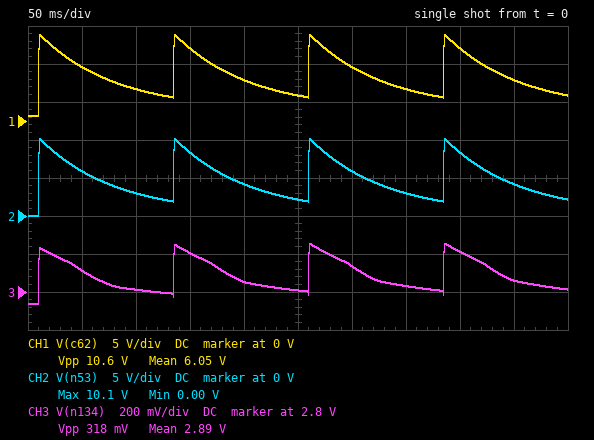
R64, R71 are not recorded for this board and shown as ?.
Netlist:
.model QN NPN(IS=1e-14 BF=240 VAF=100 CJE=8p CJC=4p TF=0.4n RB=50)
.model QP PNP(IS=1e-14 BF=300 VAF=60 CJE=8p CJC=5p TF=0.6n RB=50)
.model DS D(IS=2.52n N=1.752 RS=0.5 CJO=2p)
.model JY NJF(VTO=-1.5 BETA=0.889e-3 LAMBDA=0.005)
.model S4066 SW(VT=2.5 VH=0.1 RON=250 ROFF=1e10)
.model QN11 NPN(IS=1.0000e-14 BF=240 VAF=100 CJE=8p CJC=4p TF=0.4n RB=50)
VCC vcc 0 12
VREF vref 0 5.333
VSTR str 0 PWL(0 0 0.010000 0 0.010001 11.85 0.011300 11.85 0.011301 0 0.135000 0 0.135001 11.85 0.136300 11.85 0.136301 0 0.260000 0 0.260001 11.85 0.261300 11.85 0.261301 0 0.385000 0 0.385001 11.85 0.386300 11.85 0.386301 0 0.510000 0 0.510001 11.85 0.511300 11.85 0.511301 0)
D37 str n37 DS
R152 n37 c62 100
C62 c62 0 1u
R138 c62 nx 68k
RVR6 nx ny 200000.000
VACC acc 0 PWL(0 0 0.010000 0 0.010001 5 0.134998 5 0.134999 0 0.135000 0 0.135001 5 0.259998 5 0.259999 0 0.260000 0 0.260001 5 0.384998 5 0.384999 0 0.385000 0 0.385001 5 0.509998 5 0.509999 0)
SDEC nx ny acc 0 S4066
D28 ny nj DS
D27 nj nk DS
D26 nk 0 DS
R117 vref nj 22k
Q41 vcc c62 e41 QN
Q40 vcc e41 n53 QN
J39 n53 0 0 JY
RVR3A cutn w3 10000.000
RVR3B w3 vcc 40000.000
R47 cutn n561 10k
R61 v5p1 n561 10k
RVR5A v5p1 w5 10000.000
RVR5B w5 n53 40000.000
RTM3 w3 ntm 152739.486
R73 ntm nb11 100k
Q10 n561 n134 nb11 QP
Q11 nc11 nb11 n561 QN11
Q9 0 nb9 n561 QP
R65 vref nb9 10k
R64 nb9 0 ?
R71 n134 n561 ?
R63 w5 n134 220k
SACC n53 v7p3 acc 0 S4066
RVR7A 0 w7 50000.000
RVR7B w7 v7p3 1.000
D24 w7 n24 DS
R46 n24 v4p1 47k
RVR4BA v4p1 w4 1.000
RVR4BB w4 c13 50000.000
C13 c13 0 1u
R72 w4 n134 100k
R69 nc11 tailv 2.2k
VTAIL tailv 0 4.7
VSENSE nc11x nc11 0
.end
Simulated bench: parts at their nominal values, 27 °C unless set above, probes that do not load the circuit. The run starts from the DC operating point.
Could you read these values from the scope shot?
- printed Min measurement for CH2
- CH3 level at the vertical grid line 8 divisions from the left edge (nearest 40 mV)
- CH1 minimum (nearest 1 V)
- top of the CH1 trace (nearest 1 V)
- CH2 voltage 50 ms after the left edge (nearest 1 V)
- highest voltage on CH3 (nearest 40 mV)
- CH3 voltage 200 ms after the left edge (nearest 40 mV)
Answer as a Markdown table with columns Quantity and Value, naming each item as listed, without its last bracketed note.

| Quantity | Value |
|---|---|
| printed Min measurement for CH2 | 0.00 V |
| CH3 level at the vertical grid line 8 divisions from the left edge | 3.00 V |
| CH1 minimum | 1 V |
| top of the CH1 trace | 11 V |
| CH2 voltage 50 ms after the left edge | 6 V |
| highest voltage on CH3 | 3.04 V |
| CH3 voltage 200 ms after the left edge | 2.84 V |
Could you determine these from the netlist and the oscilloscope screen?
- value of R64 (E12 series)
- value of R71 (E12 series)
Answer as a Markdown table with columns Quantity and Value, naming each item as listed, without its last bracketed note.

| Quantity | Value |
|---|---|
| value of R64 | 6.8 kΩ |
| value of R71 | 5.6 kΩ |
